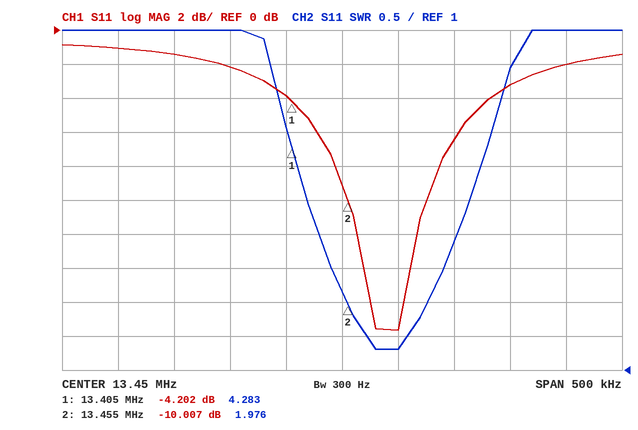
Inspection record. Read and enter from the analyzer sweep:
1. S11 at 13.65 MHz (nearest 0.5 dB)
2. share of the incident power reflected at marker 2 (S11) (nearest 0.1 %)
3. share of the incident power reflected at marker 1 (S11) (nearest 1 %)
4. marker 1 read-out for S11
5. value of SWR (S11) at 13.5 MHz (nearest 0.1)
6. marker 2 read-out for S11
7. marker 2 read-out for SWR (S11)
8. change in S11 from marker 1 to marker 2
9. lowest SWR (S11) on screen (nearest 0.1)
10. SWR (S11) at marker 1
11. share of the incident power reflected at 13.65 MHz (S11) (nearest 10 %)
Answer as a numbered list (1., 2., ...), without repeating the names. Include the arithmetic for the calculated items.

1. -2.0 dB
2. 10^(-10.007/10) ≈ 10.0 %
3. 10^(-4.202/10) ≈ 38 %
4. -4.202 dB
5. 1.3
6. -10.007 dB
7. 1.976
8. -10.007 − (-4.202) = -5.805 dB
9. 1.3
10. 4.283
11. 10^(-2/10) ≈ 63.1 %, so 60 % to the nearest 10 %
